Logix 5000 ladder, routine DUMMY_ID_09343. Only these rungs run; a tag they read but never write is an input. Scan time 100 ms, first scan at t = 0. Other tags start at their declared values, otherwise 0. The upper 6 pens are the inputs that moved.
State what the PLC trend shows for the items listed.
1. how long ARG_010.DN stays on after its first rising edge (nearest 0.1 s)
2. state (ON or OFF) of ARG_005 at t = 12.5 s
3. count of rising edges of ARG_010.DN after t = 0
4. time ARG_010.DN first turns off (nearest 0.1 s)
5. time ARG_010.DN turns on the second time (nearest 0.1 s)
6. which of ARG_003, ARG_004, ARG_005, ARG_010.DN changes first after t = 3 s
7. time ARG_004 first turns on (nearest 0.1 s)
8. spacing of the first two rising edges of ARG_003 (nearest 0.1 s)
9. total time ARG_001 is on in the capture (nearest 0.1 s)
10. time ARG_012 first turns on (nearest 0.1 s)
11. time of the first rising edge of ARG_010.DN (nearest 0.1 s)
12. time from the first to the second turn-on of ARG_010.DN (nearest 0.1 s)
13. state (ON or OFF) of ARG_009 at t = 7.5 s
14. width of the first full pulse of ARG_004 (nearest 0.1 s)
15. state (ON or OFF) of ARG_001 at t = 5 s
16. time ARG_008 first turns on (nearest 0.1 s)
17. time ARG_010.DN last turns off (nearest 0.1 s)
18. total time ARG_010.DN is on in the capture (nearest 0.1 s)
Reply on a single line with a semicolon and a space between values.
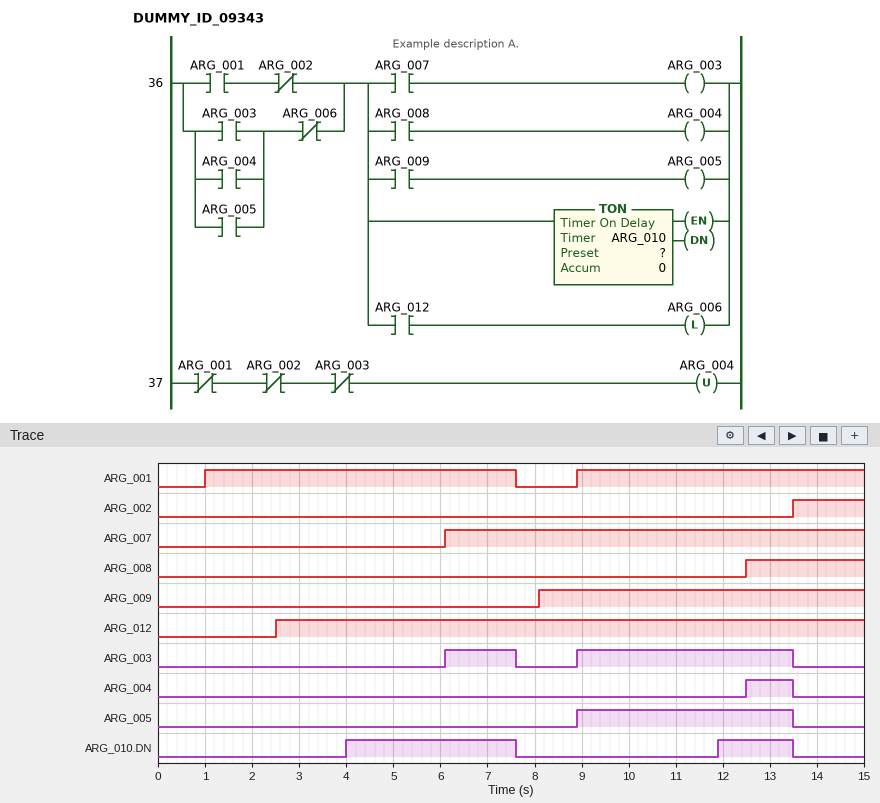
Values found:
3.6 s; ON; 2; 7.6 s; 11.9 s; ARG_010.DN; 12.5 s; 2.8 s; 12.7 s; 2.5 s; 4.0 s; 7.9 s; OFF; 1.0 s; ON; 12.5 s; 13.5 s; 5.2 s
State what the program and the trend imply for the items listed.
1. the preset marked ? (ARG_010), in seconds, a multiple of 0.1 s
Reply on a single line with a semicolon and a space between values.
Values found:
3.0 s
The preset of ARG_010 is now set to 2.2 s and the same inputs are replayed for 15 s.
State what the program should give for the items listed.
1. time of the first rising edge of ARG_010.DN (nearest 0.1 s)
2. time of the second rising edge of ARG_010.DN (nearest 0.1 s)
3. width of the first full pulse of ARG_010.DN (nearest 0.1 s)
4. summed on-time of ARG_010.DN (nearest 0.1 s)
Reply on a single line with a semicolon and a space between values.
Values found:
3.2 s; 11.1 s; 4.4 s; 6.8 s
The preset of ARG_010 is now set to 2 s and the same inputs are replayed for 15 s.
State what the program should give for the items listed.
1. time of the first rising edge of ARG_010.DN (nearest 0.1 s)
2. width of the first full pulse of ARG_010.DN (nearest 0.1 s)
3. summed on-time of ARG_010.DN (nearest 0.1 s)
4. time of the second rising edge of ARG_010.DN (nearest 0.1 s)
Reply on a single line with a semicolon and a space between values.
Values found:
3.0 s; 4.6 s; 7.2 s; 10.9 s
